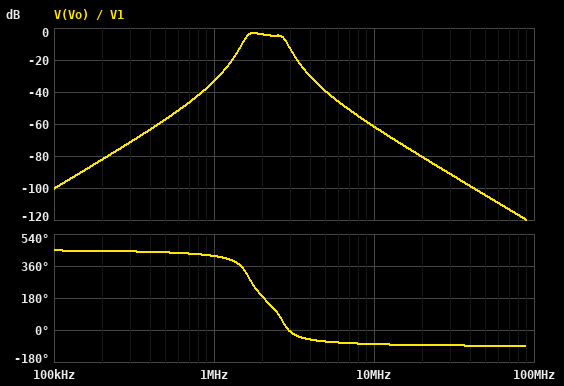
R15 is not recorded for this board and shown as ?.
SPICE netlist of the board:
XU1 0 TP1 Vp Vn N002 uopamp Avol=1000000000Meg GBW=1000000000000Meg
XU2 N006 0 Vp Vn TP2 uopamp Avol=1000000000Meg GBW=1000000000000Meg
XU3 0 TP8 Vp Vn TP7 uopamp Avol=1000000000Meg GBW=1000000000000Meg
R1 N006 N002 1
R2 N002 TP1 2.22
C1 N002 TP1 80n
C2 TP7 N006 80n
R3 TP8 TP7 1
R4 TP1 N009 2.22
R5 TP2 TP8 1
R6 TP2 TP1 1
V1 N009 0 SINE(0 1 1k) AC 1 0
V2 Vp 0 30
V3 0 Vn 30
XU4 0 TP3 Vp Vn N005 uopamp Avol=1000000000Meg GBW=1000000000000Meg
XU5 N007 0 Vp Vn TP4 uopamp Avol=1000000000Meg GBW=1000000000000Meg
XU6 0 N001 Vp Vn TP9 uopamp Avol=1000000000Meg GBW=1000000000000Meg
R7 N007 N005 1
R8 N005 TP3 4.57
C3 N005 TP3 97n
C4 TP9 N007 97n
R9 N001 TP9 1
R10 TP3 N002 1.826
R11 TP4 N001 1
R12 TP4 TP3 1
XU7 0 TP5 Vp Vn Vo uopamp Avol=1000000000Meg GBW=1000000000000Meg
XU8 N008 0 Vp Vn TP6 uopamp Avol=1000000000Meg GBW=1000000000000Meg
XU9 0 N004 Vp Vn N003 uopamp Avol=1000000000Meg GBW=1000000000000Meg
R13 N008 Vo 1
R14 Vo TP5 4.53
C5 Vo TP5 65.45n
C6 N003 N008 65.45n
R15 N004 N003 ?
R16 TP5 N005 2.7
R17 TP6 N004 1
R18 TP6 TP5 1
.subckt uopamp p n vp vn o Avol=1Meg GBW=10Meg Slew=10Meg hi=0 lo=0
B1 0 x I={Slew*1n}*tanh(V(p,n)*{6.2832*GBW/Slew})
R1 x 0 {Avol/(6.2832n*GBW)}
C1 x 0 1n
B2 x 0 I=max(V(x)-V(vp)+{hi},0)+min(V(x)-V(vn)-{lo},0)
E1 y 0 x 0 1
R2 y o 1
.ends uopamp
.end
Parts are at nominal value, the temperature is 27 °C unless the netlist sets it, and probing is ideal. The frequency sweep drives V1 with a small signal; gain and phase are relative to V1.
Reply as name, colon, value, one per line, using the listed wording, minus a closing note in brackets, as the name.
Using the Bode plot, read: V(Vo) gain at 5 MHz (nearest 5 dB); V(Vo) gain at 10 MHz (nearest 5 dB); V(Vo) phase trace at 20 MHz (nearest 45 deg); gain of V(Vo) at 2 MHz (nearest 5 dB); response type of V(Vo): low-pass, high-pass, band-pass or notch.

V(Vo) gain at 5 MHz: -40 dB
V(Vo) gain at 10 MHz: -60 dB
V(Vo) phase trace at 20 MHz: -90 deg
gain of V(Vo) at 2 MHz: -5 dB
response type of V(Vo): low-pass, high-pass, band-pass or notch: band-pass
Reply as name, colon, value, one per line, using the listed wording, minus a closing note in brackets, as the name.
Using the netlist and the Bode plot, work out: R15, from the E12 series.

R15, from the E12 series: 0.82 Ω
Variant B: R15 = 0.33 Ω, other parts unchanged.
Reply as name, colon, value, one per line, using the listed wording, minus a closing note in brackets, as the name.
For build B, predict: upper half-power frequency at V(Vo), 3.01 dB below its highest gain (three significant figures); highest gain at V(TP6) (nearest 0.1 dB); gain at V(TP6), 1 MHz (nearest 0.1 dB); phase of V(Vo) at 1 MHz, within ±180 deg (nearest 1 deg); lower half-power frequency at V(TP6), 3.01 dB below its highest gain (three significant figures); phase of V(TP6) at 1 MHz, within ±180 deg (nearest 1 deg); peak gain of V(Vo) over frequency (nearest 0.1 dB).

upper half-power frequency at V(Vo), 3.01 dB below its highest gain: 2.08 MHz
highest gain at V(TP6): -1.3 dB
gain at V(TP6), 1 MHz: -24.6 dB
phase of V(Vo) at 1 MHz, within ±180 deg: 59 deg
lower half-power frequency at V(TP6), 3.01 dB below its highest gain: 1.54 MHz
phase of V(TP6) at 1 MHz, within ±180 deg: -31 deg
peak gain of V(Vo) over frequency: -14.0 dB
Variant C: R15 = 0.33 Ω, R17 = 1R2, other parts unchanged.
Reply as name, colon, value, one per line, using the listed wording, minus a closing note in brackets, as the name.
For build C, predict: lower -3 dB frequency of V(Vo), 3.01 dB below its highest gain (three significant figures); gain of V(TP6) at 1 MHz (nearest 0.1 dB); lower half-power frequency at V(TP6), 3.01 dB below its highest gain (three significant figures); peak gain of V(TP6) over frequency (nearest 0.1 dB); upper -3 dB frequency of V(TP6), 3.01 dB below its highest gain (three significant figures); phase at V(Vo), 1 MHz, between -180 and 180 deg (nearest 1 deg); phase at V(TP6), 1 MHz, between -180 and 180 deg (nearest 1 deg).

lower -3 dB frequency of V(Vo), 3.01 dB below its highest gain: 1.56 MHz
gain of V(TP6) at 1 MHz: -24.7 dB
lower half-power frequency at V(TP6), 3.01 dB below its highest gain: 1.54 MHz
peak gain of V(TP6) over frequency: -1.6 dB
upper -3 dB frequency of V(TP6), 3.01 dB below its highest gain: 1.96 MHz
phase at V(Vo), 1 MHz, between -180 and 180 deg: 60 deg
phase at V(TP6), 1 MHz, between -180 and 180 deg: -30 deg
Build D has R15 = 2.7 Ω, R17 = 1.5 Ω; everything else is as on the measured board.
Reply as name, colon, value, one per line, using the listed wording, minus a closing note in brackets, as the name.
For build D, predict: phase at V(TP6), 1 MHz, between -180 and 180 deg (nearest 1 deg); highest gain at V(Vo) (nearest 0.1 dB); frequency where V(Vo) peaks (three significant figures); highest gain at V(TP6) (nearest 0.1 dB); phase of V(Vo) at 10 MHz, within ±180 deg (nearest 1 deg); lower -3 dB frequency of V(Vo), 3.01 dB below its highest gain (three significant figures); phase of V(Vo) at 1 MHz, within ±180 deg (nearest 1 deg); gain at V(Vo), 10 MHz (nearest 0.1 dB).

phase at V(TP6), 1 MHz, between -180 and 180 deg: -42 deg
highest gain at V(Vo): 9.7 dB
frequency where V(Vo) peaks: 1.74 MHz
highest gain at V(TP6): 7.6 dB
phase of V(Vo) at 10 MHz, within ±180 deg: -79 deg
lower -3 dB frequency of V(Vo), 3.01 dB below its highest gain: 1.59 MHz
phase of V(Vo) at 1 MHz, within ±180 deg: 48 deg
gain at V(Vo), 10 MHz: -62.0 dB
